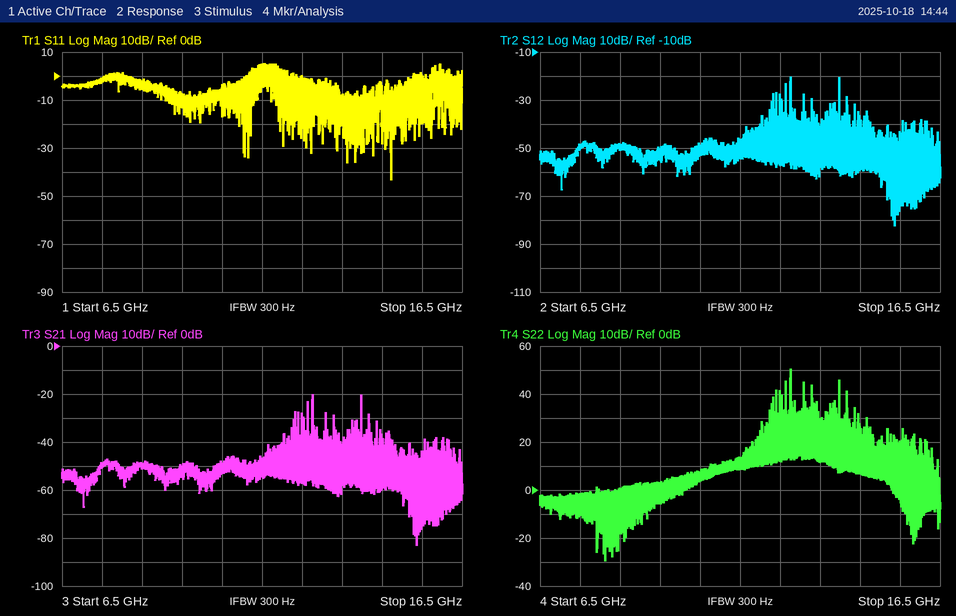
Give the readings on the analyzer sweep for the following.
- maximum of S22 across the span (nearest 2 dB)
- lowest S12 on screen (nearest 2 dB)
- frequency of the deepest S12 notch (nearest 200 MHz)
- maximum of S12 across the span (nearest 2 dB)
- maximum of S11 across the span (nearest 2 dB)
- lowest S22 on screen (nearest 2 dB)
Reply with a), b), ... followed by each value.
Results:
a) 50 dB
b) -82 dB
c) 15.4 GHz
d) -20 dB
e) 6 dB
f) -30 dB
